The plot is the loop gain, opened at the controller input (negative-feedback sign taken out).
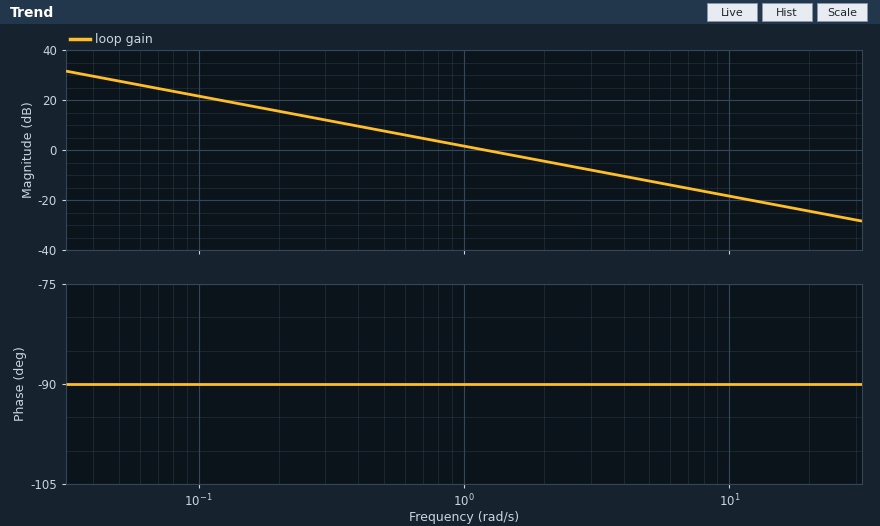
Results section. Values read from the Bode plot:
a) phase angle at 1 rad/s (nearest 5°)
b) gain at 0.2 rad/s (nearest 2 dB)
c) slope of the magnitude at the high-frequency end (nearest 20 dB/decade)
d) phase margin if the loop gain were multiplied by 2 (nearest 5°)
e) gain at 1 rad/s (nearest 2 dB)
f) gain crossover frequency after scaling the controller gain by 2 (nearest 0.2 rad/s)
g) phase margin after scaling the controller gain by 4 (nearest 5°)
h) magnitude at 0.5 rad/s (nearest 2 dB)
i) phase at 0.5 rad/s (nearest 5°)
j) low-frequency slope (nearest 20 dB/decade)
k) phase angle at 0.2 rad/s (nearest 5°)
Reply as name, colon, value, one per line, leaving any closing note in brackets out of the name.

phase angle at 1 rad/s: -90°
gain at 0.2 rad/s: 16 dB
slope of the magnitude at the high-frequency end: -20 dB/decade
phase margin if the loop gain were multiplied by 2: 90°
gain at 1 rad/s: 2 dB
gain crossover frequency after scaling the controller gain by 2: 2.4 rad/s
phase margin after scaling the controller gain by 4: 90°
magnitude at 0.5 rad/s: 8 dB
phase at 0.5 rad/s: -90°
low-frequency slope: -20 dB/decade
phase angle at 0.2 rad/s: -90°
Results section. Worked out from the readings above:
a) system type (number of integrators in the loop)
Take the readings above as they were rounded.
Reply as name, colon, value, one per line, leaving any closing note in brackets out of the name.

system type: 1
